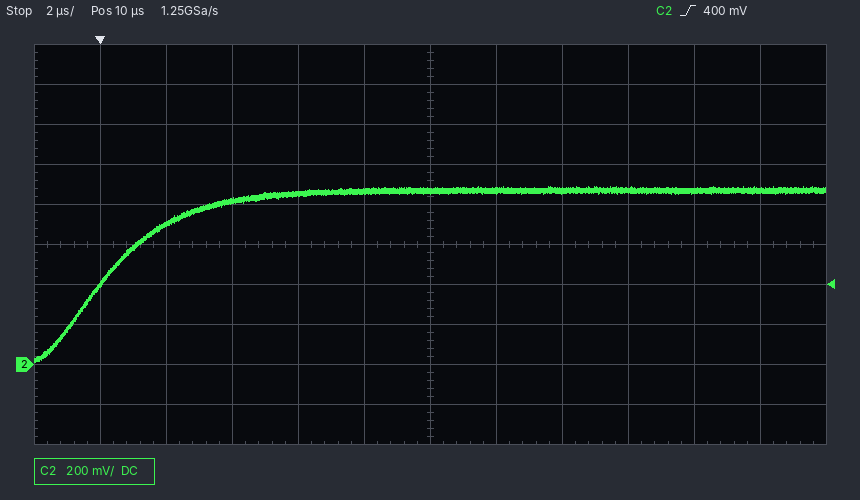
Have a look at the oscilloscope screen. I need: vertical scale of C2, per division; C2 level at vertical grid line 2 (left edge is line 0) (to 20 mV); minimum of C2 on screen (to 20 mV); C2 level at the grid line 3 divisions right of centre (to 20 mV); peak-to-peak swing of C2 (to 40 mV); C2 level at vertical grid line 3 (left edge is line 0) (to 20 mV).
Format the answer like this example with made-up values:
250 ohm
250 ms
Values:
200 mV
700 mV
20 mV
880 mV
880 mV
820 mV
